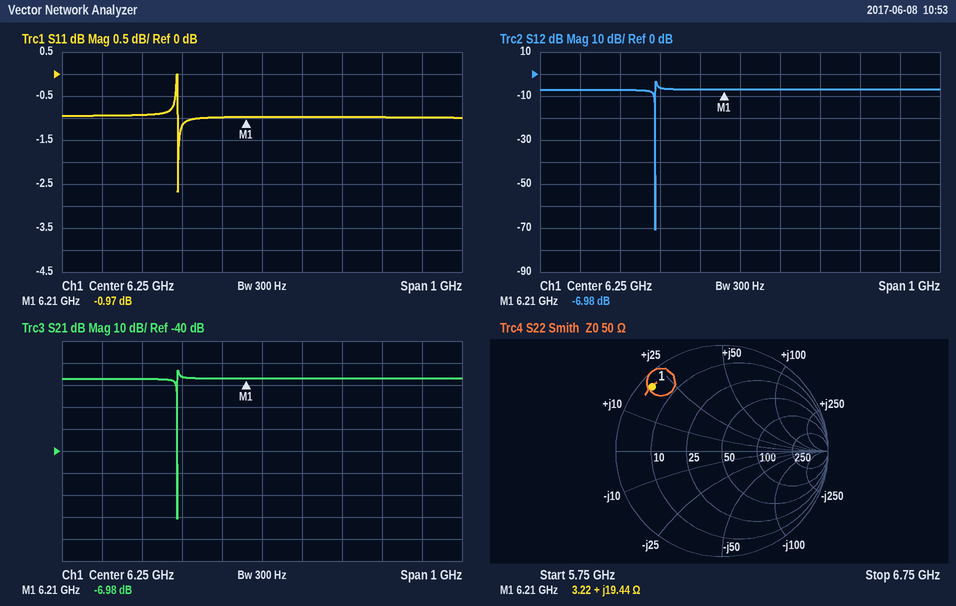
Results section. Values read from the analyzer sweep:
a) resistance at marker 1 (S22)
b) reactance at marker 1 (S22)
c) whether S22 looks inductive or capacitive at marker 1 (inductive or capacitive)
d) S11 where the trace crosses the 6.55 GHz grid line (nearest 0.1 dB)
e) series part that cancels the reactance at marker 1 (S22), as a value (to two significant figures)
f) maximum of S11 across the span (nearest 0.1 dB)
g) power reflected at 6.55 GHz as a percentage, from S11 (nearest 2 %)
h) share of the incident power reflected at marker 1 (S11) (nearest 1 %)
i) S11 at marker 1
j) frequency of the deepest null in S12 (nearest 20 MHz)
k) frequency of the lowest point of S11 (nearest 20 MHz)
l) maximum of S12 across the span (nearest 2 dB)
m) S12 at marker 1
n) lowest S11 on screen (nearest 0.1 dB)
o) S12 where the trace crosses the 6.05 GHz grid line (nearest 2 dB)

3.22 Ω
+19.44 Ω
inductive
-1.0 dB
1.3 pF
0.0 dB
80 %
80 %
-0.97 dB
6.04 GHz
6.04 GHz
-4 dB
-6.98 dB
-2.7 dB
-6 dB
